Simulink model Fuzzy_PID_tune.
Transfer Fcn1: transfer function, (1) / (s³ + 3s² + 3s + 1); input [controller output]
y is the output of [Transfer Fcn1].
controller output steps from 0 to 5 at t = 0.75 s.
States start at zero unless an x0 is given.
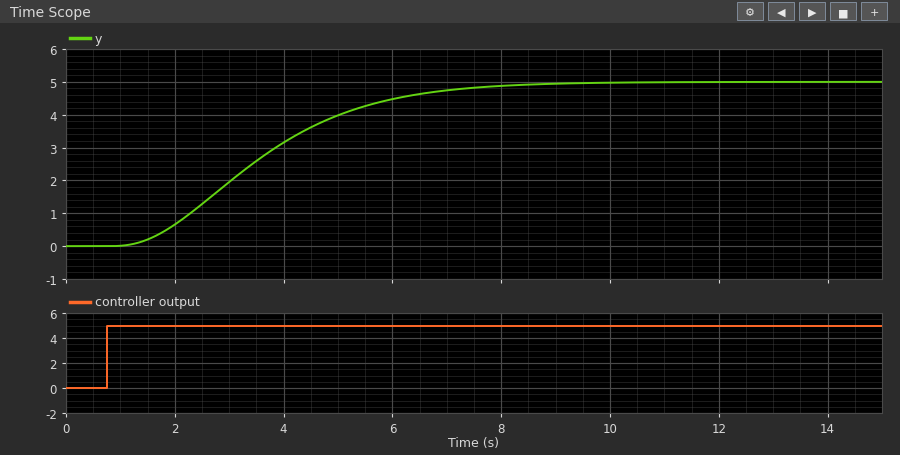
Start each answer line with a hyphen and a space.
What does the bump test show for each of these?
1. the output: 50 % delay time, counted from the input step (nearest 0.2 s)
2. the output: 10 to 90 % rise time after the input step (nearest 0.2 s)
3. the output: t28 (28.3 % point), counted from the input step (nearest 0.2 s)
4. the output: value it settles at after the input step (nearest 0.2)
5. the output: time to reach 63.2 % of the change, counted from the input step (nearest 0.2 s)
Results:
- 2.6 s
- 4.2 s
- 1.8 s
- 5.0
- 3.2 s
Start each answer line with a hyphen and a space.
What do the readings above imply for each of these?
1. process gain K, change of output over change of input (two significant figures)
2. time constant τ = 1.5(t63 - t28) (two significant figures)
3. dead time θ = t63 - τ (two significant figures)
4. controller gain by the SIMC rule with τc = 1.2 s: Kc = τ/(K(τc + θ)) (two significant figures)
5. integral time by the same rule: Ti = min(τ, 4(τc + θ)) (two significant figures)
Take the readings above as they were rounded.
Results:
- 1.0
- 2.1 s
- 1.1 s
- 0.91
- 2.1 s
